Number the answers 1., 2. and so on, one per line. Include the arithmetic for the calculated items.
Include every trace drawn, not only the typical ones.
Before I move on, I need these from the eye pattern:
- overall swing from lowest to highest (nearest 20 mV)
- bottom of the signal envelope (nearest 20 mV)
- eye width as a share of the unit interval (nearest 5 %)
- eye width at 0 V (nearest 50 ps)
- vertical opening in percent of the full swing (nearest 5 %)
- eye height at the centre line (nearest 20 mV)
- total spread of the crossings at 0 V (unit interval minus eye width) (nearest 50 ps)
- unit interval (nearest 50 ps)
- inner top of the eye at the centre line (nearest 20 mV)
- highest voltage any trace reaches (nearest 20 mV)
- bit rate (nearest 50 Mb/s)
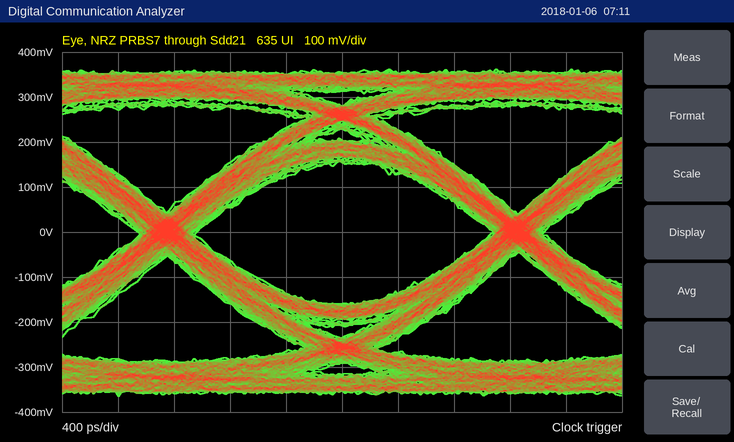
1. 720 mV
2. -360 mV
3. 2.10 ns / 2.50 ns ≈ 84.0 %, so 85 % to the nearest 5 %
4. 2.10 ns
5. 320 mV / 720 mV ≈ 44.4 %, so 45 % to the nearest 5 %
6. 320 mV
7. 400 ps
8. 2.50 ns
9. 160 mV
10. 360 mV
11. 400 Mb/s
